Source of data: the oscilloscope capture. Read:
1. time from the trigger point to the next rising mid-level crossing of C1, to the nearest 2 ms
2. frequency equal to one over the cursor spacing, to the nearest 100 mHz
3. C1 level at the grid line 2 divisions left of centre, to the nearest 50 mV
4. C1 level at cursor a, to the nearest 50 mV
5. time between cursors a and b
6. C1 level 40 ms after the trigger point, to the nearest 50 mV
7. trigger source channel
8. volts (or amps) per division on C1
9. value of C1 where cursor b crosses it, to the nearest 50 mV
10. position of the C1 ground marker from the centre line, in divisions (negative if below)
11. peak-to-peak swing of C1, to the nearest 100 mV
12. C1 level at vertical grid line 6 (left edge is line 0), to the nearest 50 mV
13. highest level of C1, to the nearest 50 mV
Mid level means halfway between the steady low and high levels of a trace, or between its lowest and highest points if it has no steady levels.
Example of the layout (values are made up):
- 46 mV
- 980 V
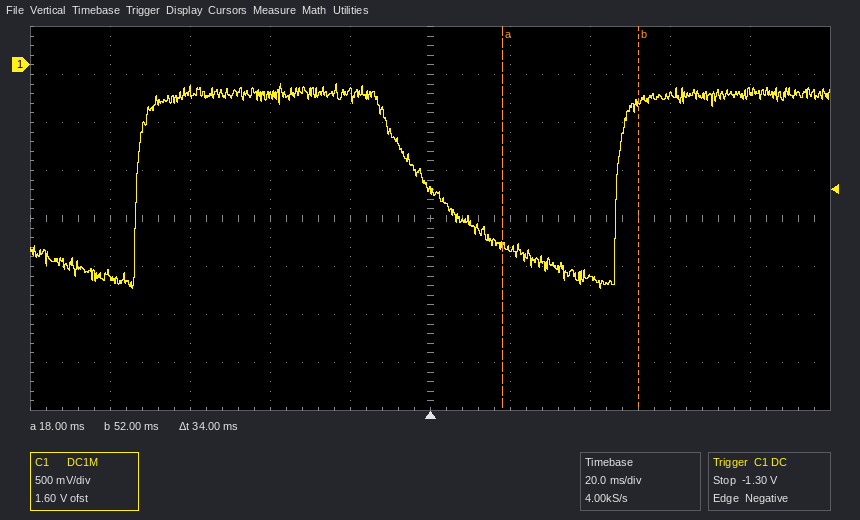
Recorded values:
- 46 ms
- 29.4 Hz
- -300 mV
- -1.90 V
- 34 ms
- -2.20 V
- C1
- 500 mV
- -400 mV
- +3.2 div
- 2.10 V
- -1.90 V
- -200 mV
